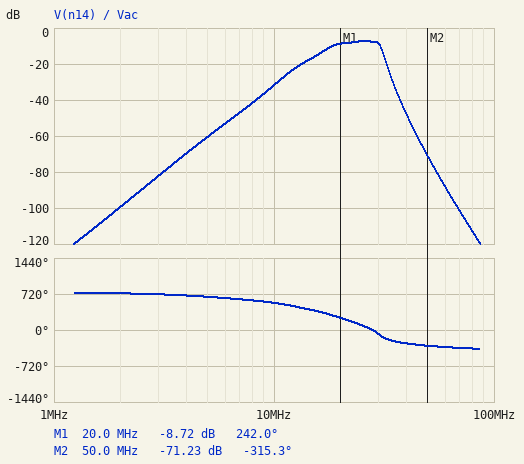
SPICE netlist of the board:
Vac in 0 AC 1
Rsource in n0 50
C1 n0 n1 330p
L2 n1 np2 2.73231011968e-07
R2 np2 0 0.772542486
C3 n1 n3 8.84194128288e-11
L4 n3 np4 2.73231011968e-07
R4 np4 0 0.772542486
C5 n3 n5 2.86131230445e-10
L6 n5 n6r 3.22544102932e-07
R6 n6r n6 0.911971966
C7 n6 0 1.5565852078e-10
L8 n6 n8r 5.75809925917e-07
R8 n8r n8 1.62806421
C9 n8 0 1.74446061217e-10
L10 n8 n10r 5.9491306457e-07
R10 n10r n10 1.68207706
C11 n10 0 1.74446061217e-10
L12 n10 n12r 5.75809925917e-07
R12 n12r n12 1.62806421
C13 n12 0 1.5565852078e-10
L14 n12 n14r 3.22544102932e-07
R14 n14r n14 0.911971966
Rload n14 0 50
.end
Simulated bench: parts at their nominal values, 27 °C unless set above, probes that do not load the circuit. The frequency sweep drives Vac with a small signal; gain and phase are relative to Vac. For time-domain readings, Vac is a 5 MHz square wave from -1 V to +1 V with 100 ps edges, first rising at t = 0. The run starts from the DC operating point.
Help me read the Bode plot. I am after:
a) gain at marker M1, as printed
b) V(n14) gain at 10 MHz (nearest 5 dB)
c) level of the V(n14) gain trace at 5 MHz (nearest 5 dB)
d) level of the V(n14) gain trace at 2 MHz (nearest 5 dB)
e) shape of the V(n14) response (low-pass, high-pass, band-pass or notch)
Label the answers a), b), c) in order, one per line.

a) -8.72 dB
b) -30 dB
c) -60 dB
d) -100 dB
e) band-pass
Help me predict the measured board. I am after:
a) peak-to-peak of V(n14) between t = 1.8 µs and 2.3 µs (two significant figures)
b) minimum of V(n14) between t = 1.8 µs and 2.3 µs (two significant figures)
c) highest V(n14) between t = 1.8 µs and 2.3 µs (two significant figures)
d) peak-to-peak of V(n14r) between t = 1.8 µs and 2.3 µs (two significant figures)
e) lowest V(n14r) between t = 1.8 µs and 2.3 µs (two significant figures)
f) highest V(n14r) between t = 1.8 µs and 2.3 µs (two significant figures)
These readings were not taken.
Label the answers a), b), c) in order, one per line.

a) 350 mV
b) -180 mV
c) 180 mV
d) 360 mV
e) -180 mV
f) 180 mV
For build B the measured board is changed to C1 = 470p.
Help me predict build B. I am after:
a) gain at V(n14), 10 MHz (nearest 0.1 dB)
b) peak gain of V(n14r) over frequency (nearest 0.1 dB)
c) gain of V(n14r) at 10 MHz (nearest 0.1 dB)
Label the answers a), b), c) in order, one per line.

a) -30.9 dB
b) -7.2 dB
c) -30.7 dB
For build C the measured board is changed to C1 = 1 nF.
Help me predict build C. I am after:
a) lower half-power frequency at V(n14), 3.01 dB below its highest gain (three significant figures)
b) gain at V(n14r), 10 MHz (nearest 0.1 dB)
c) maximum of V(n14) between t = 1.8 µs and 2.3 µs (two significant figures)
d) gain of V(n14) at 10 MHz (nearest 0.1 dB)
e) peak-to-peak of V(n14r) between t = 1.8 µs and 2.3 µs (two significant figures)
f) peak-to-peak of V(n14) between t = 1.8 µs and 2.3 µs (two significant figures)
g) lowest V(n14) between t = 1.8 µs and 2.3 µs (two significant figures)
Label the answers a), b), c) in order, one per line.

a) 18.8 MHz
b) -30.4 dB
c) 170 mV
d) -30.6 dB
e) 350 mV
f) 340 mV
g) -170 mV
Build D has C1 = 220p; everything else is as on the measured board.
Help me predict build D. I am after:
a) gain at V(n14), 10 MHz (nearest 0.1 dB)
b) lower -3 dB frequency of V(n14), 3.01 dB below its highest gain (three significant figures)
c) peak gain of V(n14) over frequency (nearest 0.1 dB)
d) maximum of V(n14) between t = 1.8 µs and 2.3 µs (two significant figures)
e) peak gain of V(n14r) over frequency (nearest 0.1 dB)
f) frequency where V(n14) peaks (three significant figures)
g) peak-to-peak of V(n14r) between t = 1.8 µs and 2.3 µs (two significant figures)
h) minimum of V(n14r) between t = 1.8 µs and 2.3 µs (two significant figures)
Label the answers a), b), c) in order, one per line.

a) -33.7 dB
b) 18.0 MHz
c) -7.2 dB
d) 170 mV
e) -7.0 dB
f) 25.6 MHz
g) 350 mV
h) -170 mV
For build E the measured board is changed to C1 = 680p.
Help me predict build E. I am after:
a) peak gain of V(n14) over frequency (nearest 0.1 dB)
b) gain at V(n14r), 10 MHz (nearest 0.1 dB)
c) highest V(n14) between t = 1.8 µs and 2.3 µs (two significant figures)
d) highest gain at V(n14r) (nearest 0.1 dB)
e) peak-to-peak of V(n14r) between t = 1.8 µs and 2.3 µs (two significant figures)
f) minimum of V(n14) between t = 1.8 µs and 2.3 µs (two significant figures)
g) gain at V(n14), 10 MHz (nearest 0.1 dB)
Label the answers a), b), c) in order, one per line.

a) -7.4 dB
b) -30.4 dB
c) 170 mV
d) -7.3 dB
e) 350 mV
f) -170 mV
g) -30.6 dB
